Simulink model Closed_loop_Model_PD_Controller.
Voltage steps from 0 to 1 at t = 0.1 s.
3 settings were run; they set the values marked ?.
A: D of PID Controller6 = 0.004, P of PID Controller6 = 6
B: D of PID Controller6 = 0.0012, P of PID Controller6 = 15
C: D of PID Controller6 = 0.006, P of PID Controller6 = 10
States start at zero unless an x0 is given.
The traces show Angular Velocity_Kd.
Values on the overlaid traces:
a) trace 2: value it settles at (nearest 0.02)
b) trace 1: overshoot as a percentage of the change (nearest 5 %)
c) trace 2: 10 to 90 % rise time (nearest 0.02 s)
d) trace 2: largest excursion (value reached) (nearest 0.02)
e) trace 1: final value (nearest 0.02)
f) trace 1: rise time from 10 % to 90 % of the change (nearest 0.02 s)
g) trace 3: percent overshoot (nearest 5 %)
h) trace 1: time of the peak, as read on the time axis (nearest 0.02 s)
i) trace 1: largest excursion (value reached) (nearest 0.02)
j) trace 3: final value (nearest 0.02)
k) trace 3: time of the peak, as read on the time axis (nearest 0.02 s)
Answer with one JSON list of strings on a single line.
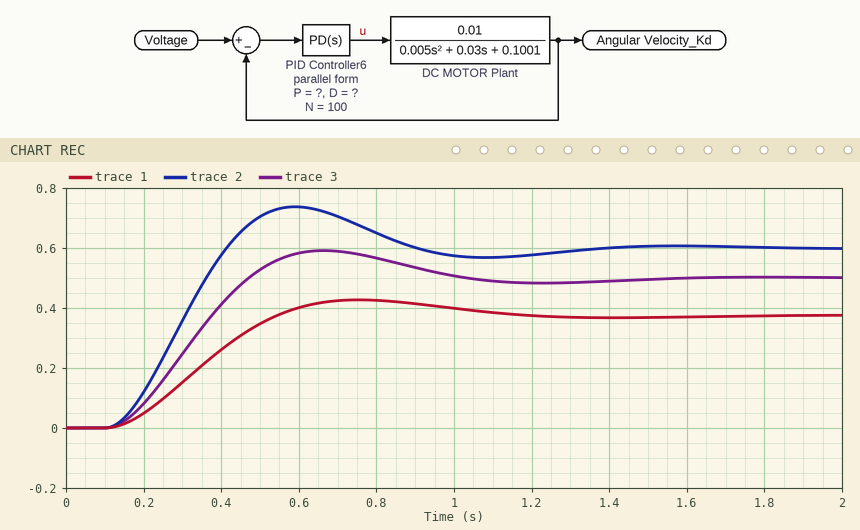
["0.60", "15 %", "0.22 s", "0.74", "0.38", "0.30 s", "20 %", "0.76 s", "0.42", "0.50", "0.66 s"]
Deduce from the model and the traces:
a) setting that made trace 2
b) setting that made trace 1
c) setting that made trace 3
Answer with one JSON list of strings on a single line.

["B", "A", "C"]
